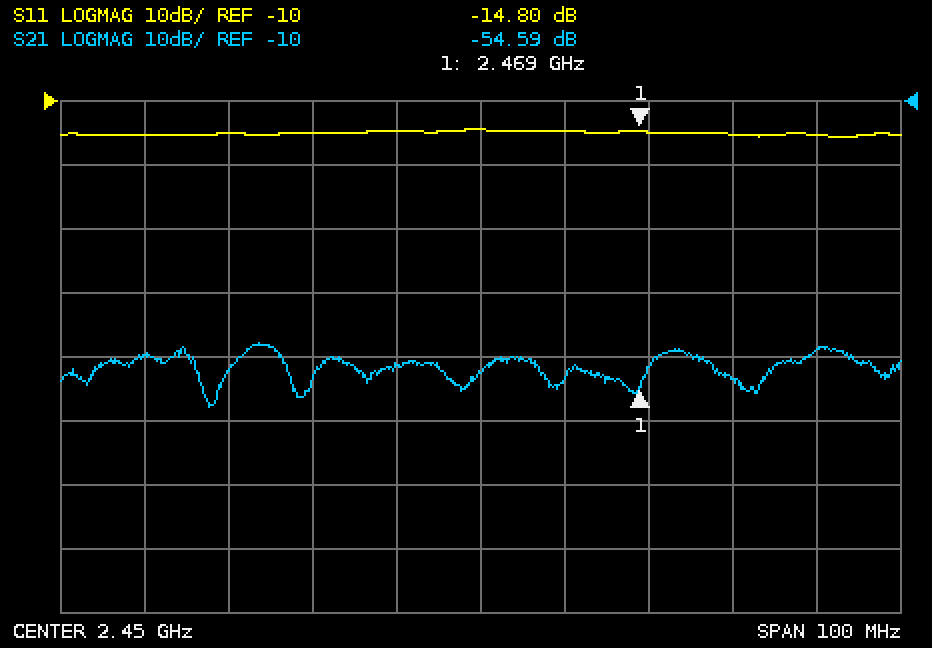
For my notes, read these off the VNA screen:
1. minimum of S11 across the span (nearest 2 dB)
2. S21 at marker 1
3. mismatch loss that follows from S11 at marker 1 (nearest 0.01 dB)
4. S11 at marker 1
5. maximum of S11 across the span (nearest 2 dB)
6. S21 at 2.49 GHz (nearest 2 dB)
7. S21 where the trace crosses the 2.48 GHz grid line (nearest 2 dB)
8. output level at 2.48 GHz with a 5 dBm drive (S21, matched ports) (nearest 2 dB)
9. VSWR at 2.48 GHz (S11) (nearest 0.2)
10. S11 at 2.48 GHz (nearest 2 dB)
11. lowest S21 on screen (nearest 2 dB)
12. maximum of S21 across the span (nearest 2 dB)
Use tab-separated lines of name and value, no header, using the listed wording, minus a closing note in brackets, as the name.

minimum of S11 across the span	-16 dB
S21 at marker 1	-54.59 dB
mismatch loss that follows from S11 at marker 1	0.15 dB
S11 at marker 1	-14.80 dB
maximum of S11 across the span	-14 dB
S21 at 2.49 GHz	-48 dB
S21 where the trace crosses the 2.48 GHz grid line	-54 dB
output level at 2.48 GHz with a 5 dBm drive (S21, matched ports)	-48 dBm
VSWR at 2.48 GHz (S11)	1.4
S11 at 2.48 GHz	-16 dB
lowest S21 on screen	-58 dB
maximum of S21 across the span	-48 dB
